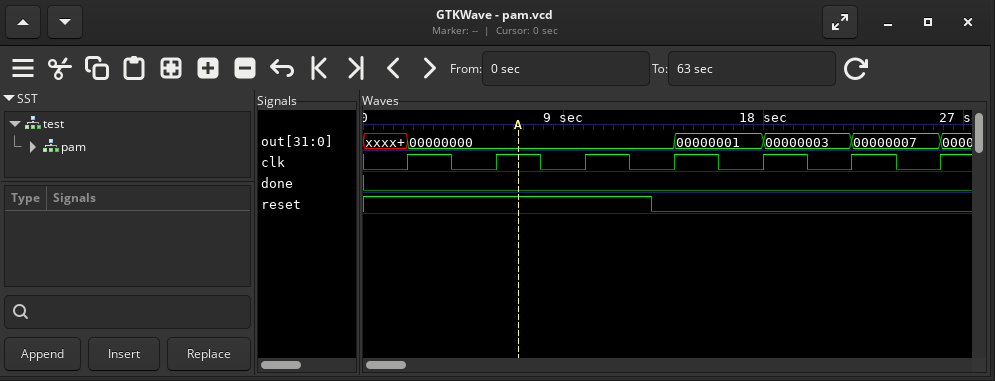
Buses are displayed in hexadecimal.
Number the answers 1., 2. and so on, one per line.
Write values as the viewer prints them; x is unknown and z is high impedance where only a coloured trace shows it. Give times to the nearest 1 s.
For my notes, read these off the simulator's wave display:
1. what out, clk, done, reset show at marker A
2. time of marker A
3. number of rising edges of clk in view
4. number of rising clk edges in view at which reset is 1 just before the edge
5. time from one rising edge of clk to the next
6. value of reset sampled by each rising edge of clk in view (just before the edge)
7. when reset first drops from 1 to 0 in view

1. out=00000000, clk=1, done=0, reset=1
2. 7 s
3. 7
4. 3
5. 4 s
6. 1 1 1 0 0 0 0
7. 13 s
